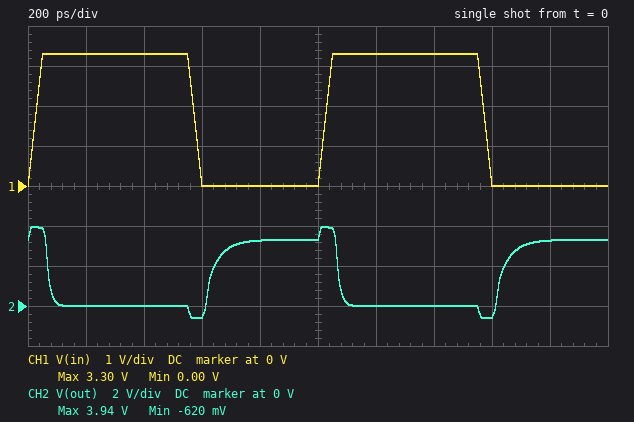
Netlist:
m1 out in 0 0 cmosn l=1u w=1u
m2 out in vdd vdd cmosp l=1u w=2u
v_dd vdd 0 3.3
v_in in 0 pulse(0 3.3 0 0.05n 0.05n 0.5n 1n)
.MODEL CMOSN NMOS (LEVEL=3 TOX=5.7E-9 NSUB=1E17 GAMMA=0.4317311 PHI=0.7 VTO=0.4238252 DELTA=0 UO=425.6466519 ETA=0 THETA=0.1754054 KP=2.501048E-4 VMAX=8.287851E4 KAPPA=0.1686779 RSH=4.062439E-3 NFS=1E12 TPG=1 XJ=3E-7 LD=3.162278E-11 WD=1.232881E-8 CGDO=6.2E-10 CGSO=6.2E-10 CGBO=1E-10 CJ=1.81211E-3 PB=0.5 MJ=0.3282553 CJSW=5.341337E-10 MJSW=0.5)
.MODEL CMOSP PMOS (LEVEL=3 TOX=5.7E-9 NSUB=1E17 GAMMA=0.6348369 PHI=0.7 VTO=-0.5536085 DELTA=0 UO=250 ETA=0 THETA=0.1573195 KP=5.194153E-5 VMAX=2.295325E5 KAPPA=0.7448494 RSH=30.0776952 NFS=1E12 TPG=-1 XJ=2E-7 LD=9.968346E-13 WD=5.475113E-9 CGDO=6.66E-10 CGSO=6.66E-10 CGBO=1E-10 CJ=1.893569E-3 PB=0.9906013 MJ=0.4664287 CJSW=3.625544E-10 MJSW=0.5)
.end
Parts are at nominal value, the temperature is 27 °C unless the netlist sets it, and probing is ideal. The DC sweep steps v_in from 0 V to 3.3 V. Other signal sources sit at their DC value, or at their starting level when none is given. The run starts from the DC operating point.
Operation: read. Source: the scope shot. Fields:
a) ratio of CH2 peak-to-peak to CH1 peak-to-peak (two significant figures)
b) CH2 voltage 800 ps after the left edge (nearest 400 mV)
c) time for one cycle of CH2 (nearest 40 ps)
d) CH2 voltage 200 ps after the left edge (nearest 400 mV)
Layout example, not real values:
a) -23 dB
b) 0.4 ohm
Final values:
a) 1.4
b) 3.2 V
c) 1.00 ns
d) 0 V
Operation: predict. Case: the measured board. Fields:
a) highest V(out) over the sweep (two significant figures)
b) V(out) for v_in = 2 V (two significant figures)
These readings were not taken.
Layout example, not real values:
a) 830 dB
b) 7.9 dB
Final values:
a) 3.3 V
b) 81 mV
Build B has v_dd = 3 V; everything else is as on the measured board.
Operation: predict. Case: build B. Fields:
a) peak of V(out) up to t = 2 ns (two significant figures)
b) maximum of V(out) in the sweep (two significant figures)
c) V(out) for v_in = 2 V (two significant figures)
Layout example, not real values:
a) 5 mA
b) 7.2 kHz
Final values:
a) 3.6 V
b) 3.0 V
c) 32 mV
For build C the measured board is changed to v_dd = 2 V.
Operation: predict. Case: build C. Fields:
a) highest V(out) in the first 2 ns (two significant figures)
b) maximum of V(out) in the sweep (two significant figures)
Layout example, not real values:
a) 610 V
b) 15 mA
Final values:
a) 2.6 V
b) 2.0 V
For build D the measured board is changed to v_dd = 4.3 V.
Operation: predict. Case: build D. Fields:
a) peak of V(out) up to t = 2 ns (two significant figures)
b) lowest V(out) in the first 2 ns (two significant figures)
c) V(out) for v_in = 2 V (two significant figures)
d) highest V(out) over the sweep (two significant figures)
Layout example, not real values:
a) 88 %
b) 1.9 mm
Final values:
a) 4.9 V
b) -590 mV
c) 460 mV
d) 4.3 V
